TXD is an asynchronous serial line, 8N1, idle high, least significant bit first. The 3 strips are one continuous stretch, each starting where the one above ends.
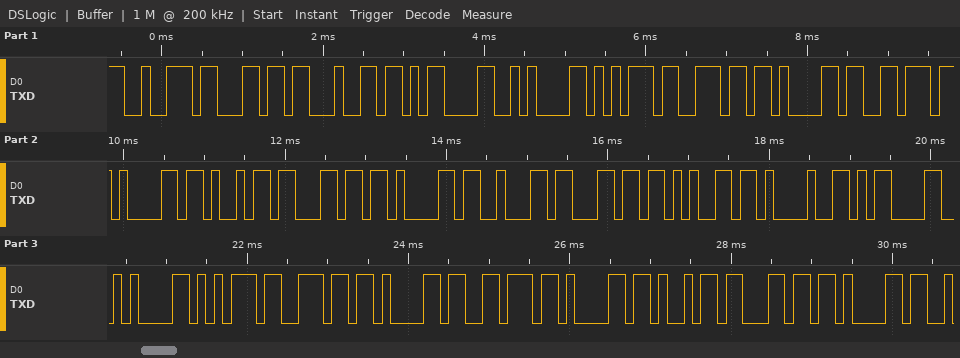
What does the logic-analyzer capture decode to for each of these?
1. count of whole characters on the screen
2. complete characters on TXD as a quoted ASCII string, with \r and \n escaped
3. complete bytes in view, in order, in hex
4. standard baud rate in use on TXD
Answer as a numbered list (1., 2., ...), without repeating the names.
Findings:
1. 27
2. "rld\r\nunavailable!\r\nunavaila"
3. 72 6C 64 0D 0A 75 6E 61 76 61 69 6C 61 62 6C 65 21 0D 0A 75 6E 61 76 61 69 6C 61
4. 9600 baud
